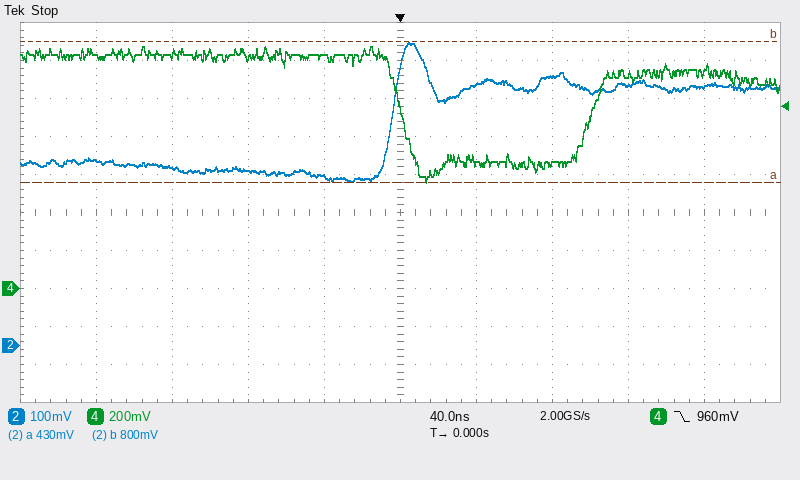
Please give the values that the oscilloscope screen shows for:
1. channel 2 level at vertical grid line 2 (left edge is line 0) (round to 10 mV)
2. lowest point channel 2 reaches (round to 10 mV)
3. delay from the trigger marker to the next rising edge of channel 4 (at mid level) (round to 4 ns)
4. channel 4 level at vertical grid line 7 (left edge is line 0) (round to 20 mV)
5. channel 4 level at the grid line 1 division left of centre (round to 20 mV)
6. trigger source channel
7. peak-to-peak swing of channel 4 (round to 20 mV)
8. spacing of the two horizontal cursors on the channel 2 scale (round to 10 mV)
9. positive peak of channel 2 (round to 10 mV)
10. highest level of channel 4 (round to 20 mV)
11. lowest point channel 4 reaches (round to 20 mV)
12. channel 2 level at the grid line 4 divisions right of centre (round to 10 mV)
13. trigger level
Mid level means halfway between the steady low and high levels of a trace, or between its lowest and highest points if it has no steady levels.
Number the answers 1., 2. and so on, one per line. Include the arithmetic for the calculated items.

1. 470 mV
2. 430 mV
3. 100 ns
4. 660 mV
5. 1.22 V
6. channel 4
7. 1.28 V − (560 mV) = 720 mV
8. 370 mV
9. 800 mV
10. 1.28 V
11. 560 mV
12. 680 mV
13. 960 mV
